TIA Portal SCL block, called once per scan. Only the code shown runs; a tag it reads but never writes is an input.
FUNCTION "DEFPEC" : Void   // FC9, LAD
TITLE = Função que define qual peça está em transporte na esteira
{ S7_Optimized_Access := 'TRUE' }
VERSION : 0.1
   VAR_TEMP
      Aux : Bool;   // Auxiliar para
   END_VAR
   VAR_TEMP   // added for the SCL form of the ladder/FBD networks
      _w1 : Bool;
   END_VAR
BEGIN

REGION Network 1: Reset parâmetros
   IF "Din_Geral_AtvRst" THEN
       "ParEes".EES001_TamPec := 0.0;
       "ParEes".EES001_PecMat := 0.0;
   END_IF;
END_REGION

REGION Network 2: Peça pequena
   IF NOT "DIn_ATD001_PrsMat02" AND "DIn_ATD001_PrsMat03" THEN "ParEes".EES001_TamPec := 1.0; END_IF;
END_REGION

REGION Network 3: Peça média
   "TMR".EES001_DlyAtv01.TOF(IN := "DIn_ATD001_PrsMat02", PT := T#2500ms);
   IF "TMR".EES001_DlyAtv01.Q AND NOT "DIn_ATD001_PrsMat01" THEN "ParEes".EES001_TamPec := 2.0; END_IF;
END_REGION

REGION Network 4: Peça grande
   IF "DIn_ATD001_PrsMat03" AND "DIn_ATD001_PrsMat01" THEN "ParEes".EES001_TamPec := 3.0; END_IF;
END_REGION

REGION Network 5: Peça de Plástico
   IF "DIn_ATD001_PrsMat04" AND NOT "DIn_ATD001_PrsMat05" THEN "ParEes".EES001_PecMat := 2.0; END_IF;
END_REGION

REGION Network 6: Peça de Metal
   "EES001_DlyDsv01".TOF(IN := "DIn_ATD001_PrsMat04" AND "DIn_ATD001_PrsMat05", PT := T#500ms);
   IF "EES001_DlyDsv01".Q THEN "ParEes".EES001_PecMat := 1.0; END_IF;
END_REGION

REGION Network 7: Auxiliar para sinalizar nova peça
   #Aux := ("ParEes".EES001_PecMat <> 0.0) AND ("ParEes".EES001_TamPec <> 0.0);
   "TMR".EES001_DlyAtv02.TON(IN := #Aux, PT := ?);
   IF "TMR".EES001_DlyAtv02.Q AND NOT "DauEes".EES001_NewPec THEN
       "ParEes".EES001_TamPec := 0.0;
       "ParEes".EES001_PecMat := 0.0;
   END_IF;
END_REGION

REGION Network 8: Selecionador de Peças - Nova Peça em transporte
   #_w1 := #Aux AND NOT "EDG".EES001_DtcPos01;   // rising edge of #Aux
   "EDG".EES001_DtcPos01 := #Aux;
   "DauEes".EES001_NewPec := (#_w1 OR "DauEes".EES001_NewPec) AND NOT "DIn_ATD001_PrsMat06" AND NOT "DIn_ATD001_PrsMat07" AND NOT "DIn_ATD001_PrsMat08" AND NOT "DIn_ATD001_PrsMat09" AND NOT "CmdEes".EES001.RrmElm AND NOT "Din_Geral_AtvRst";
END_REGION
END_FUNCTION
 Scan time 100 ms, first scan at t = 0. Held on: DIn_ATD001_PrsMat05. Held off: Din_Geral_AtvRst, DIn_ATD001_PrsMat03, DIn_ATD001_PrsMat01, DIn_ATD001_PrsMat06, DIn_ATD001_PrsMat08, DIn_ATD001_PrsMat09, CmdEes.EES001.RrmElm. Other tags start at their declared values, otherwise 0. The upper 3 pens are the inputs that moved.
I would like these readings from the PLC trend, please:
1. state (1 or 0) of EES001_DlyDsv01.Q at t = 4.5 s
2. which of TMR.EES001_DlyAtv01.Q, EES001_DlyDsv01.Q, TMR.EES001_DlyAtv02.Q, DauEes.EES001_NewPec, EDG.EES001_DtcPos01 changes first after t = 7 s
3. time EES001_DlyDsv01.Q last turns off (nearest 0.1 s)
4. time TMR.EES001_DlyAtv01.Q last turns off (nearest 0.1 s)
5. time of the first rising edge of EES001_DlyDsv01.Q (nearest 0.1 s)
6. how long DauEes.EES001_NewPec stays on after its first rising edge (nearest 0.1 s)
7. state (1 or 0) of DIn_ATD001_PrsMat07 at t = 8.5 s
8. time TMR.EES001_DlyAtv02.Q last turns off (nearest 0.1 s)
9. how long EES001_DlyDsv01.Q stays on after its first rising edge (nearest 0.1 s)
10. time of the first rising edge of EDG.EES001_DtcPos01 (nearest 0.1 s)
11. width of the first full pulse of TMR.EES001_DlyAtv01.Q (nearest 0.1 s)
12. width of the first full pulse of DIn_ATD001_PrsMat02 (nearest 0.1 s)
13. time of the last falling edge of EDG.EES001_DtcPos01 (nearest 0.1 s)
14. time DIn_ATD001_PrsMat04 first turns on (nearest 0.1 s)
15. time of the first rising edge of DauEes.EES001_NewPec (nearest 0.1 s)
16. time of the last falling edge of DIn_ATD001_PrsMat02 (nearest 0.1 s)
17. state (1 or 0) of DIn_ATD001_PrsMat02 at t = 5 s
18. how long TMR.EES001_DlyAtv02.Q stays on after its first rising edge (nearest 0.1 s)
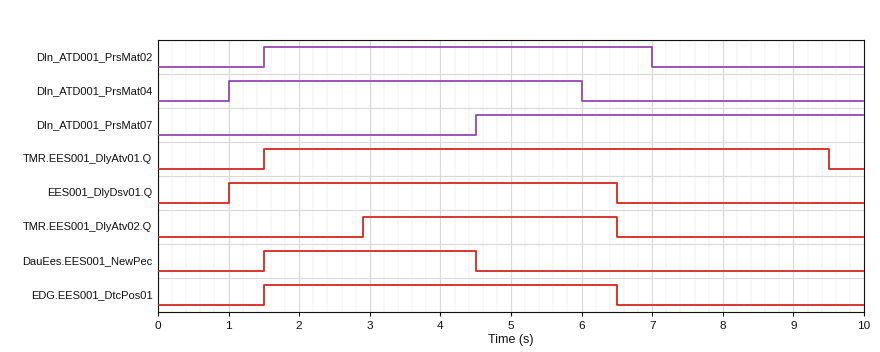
1
TMR.EES001_DlyAtv01.Q
6.5 s
9.5 s
1.0 s
3.0 s
1
6.5 s
5.5 s
1.5 s
8.0 s
5.5 s
6.5 s
1.0 s
1.5 s
7.0 s
1
3.6 s
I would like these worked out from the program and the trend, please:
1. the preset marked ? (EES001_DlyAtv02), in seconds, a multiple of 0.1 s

1.4 s
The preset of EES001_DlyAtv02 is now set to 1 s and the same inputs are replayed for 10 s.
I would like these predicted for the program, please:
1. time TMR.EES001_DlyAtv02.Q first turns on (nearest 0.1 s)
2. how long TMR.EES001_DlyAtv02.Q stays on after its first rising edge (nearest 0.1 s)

2.5 s
4.0 s
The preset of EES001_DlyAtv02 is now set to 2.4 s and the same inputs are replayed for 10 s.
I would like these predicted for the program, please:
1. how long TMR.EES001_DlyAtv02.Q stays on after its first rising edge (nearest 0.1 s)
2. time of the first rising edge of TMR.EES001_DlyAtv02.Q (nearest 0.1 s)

2.6 s
3.9 s
